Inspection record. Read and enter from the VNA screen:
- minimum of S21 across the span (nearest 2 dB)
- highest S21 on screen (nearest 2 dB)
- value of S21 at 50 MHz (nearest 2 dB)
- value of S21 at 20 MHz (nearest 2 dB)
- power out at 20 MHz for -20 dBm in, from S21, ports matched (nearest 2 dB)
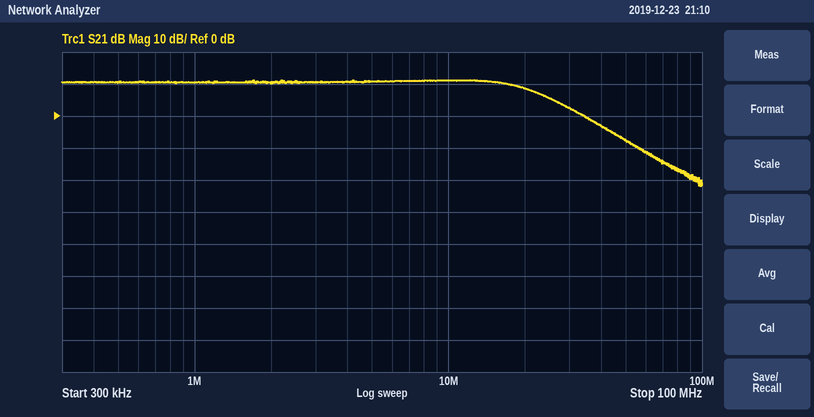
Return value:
-22 dB
12 dB
-8 dB
8 dB
-12 dBm
